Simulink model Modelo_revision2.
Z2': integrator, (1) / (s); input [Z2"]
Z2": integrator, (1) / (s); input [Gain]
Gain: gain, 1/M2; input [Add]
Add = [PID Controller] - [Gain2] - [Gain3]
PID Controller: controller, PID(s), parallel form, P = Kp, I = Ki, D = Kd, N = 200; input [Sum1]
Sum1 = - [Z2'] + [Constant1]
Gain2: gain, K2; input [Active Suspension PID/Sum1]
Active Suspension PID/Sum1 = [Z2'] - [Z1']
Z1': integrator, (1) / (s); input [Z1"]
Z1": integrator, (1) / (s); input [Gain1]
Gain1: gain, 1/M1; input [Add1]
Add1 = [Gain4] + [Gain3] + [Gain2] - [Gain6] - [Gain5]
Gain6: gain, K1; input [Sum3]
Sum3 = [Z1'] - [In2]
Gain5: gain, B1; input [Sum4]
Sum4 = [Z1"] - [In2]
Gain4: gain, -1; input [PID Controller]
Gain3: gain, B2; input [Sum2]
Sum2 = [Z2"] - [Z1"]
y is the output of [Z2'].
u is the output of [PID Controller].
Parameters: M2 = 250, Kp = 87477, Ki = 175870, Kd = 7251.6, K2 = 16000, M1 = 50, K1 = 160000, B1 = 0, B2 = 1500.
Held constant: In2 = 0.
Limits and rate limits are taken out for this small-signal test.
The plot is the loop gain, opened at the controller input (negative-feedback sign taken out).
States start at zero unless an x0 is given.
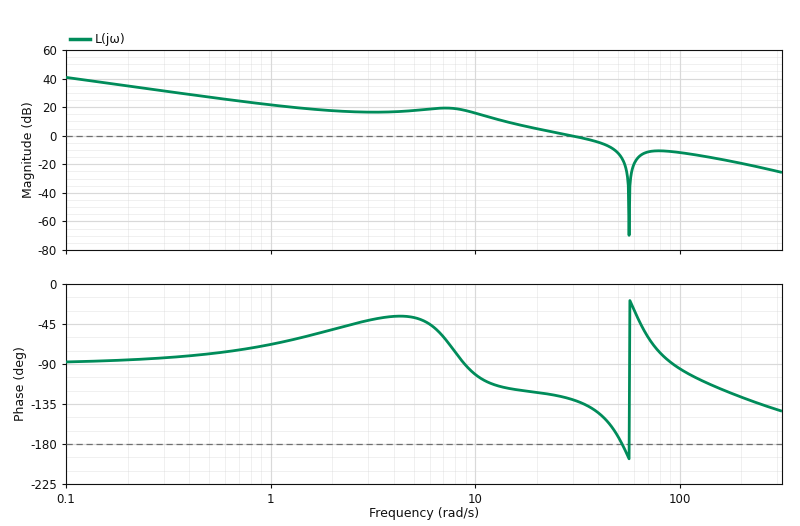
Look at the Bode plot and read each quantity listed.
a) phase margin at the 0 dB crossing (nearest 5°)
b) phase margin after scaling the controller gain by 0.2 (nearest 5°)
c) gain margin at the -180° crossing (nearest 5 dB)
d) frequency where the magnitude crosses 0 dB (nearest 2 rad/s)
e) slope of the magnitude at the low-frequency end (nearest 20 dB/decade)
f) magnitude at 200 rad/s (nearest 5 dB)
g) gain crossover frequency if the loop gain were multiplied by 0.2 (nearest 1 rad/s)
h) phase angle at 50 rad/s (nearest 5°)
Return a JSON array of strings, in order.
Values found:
["50°", "70°", "15 dB", "30 rad/s", "-20 dB/decade", "-20 dB", "11 rad/s", "-170°"]
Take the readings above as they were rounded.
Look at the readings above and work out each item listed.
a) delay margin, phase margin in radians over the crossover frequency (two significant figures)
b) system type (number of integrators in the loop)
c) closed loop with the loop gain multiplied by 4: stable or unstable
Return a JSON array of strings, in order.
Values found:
["0.029 s", "1", "stable"]
